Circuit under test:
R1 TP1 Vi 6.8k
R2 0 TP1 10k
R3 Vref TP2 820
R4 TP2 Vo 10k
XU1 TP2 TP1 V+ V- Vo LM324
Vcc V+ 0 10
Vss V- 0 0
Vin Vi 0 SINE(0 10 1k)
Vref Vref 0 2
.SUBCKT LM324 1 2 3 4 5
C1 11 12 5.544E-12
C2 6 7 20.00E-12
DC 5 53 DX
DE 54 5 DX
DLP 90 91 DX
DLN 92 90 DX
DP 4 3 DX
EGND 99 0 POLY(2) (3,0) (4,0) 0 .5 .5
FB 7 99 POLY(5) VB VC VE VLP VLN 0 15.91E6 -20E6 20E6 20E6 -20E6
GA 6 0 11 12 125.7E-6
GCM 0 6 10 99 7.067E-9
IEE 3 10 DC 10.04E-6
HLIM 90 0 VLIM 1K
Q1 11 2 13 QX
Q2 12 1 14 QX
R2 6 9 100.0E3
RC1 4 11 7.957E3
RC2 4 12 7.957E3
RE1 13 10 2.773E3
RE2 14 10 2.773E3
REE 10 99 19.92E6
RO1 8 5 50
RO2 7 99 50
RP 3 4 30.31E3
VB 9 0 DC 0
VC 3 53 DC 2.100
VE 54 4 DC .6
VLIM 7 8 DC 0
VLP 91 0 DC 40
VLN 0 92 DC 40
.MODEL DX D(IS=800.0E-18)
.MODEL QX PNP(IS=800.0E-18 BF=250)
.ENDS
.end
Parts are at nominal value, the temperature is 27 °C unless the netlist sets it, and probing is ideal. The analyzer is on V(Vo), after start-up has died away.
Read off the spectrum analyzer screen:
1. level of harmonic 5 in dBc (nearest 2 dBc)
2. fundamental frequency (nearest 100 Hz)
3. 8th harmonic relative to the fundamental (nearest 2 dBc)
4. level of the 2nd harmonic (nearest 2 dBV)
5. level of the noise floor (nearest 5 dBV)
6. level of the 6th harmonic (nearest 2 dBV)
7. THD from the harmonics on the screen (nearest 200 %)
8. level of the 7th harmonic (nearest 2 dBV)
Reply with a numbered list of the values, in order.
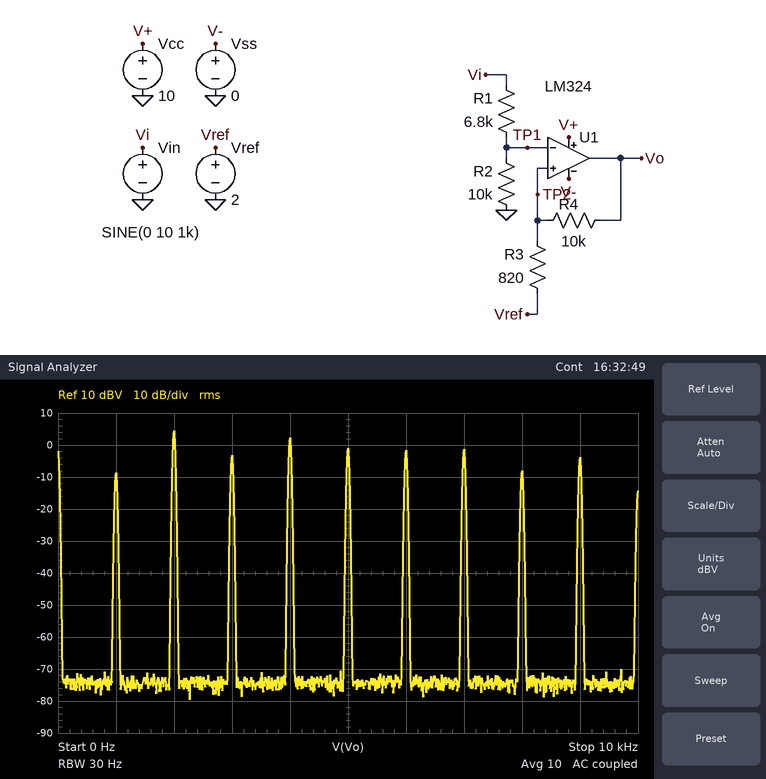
1. 8 dBc
2. 1.0 kHz
3. 0 dBc
4. 4 dBV
5. -75 dBV
6. -2 dBV
7. 800 %
8. -2 dBV
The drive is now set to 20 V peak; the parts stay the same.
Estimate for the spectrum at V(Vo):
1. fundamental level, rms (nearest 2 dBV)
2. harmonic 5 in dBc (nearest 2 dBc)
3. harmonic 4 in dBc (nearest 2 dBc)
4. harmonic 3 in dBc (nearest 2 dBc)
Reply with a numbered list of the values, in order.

1. -14 dBV
2. 4 dBc
3. 12 dBc
4. 2 dBc
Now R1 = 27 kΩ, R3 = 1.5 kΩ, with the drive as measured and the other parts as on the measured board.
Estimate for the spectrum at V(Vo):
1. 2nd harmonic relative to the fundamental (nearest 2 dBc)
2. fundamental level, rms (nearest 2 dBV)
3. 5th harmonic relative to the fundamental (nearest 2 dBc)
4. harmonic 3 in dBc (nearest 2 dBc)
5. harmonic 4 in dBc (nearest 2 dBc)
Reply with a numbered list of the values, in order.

1. -12 dBc
2. 12 dBV
3. -24 dBc
4. -12 dBc
5. -14 dBc
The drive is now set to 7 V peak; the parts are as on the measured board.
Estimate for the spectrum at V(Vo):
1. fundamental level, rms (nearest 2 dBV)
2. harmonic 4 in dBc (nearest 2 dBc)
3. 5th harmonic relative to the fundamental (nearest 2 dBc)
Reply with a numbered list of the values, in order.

1. -4 dBV
2. 6 dBc
3. 6 dBc
